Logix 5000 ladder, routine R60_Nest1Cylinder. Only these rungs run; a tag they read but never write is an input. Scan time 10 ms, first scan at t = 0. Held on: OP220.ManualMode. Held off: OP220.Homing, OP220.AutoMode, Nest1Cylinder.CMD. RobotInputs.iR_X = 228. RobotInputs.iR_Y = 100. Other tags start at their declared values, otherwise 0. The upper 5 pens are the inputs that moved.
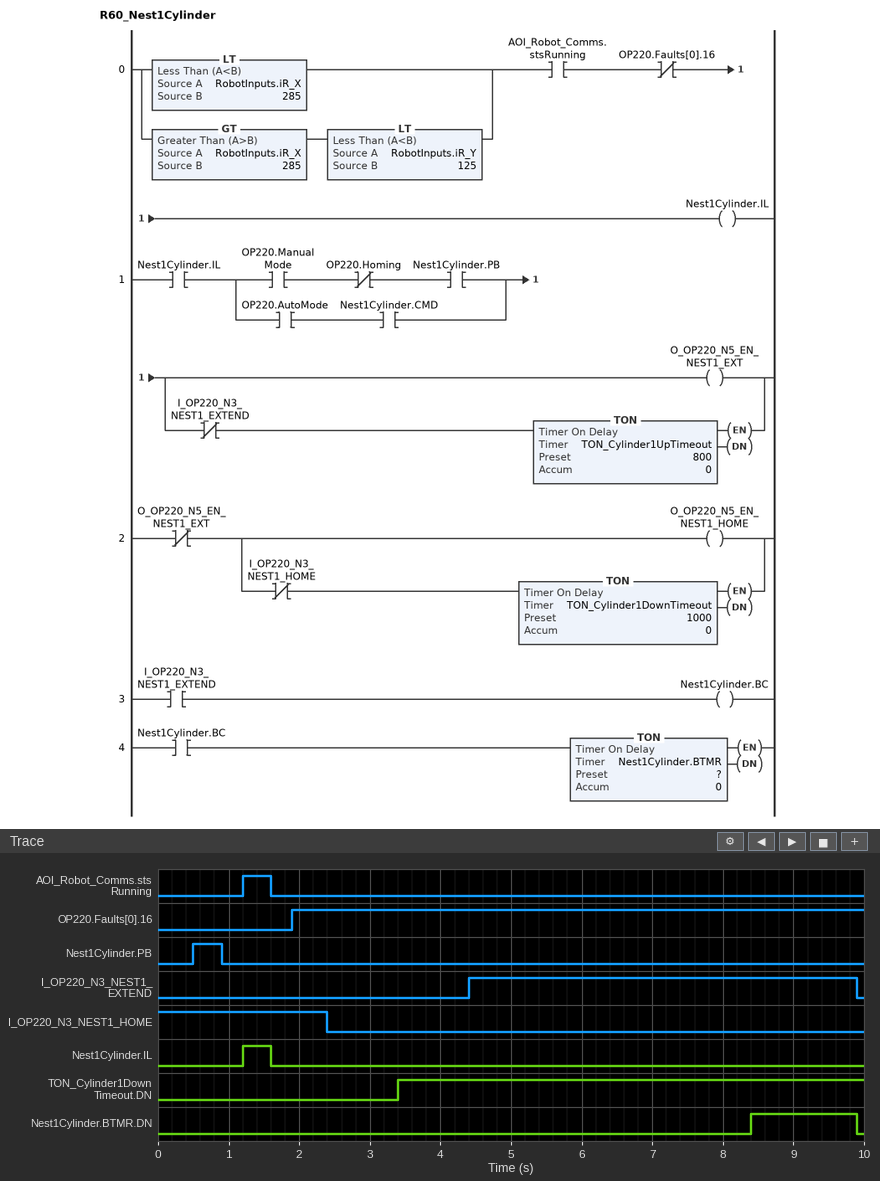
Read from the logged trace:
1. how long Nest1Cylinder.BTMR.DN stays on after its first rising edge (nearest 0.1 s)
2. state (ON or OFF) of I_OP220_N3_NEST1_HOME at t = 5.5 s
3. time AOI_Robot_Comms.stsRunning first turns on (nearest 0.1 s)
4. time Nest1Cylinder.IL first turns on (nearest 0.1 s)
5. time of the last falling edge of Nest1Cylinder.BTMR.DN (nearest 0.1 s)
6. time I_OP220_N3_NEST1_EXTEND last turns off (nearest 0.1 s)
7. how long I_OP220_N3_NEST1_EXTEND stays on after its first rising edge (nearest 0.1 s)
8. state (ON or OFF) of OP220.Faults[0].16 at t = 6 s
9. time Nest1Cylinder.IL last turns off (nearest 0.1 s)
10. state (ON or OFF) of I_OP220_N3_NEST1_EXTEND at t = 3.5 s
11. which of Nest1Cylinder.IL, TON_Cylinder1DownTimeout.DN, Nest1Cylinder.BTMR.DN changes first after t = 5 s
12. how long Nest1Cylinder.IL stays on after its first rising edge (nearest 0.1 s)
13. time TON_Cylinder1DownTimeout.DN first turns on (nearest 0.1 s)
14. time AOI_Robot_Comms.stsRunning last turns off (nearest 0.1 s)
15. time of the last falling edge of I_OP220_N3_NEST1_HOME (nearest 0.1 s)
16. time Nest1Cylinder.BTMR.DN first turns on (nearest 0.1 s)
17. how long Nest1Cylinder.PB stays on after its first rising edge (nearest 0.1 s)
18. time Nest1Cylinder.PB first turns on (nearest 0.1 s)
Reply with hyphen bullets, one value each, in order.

- 1.5 s
- OFF
- 1.2 s
- 1.2 s
- 9.9 s
- 9.9 s
- 5.5 s
- ON
- 1.6 s
- OFF
- Nest1Cylinder.BTMR.DN
- 0.4 s
- 3.4 s
- 1.6 s
- 2.4 s
- 8.4 s
- 0.4 s
- 0.5 s
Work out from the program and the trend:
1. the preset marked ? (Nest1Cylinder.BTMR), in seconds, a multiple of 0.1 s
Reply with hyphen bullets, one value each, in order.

- 4.0 s
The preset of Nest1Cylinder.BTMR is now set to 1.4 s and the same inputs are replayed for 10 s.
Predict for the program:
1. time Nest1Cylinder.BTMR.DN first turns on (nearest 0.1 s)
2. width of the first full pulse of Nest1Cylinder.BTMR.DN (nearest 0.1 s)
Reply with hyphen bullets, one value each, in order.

- 5.8 s
- 4.1 s
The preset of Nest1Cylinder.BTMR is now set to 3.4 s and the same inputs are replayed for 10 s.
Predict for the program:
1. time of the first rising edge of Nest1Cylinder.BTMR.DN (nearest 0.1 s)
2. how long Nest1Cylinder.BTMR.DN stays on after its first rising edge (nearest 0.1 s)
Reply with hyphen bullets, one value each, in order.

- 7.8 s
- 2.1 s
